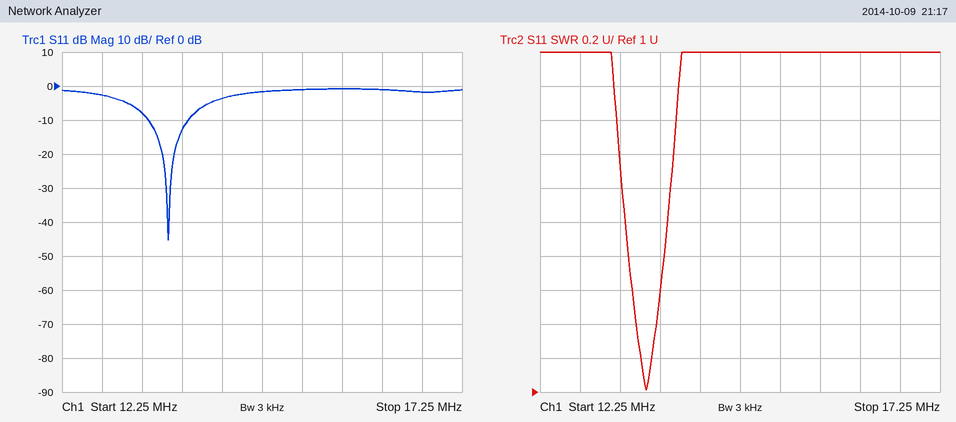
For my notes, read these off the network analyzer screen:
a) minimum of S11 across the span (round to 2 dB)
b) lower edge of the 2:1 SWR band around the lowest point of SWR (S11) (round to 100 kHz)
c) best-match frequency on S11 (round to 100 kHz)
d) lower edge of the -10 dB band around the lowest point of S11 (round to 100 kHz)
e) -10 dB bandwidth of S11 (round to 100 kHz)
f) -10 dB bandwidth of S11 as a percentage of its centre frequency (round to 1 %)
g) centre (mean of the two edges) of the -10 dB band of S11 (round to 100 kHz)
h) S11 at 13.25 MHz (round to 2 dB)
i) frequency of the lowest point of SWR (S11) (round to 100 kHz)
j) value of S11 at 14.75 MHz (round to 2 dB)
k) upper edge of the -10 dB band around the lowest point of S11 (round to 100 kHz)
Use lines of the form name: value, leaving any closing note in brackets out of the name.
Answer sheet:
minimum of S11 across the span: -46 dB
lower edge of the 2:1 SWR band around the lowest point of SWR (S11): 13.3 MHz
best-match frequency on S11: 13.6 MHz
lower edge of the -10 dB band around the lowest point of S11: 13.3 MHz
-10 dB bandwidth of S11: 500 kHz
-10 dB bandwidth of S11 as a percentage of its centre frequency: 4 %
centre (mean of the two edges) of the -10 dB band of S11: 13.6 MHz
S11 at 13.25 MHz: -8 dB
frequency of the lowest point of SWR (S11): 13.6 MHz
value of S11 at 14.75 MHz: -2 dB
upper edge of the -10 dB band around the lowest point of S11: 13.8 MHz
